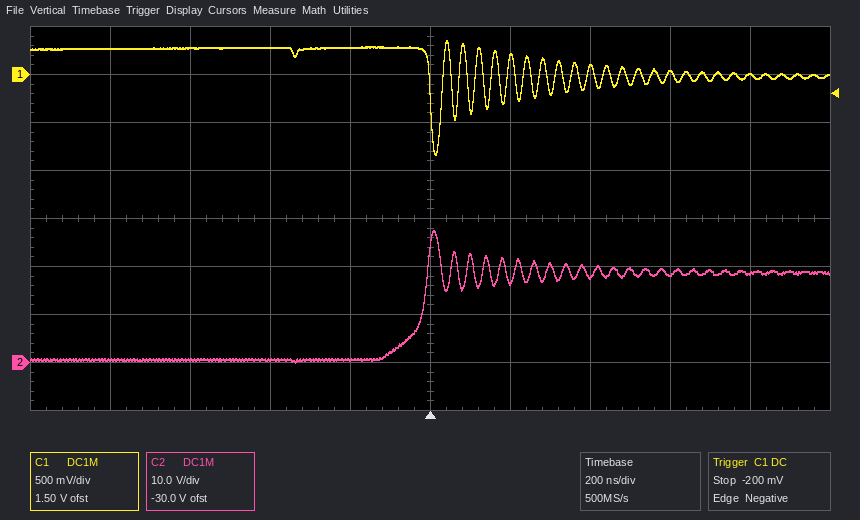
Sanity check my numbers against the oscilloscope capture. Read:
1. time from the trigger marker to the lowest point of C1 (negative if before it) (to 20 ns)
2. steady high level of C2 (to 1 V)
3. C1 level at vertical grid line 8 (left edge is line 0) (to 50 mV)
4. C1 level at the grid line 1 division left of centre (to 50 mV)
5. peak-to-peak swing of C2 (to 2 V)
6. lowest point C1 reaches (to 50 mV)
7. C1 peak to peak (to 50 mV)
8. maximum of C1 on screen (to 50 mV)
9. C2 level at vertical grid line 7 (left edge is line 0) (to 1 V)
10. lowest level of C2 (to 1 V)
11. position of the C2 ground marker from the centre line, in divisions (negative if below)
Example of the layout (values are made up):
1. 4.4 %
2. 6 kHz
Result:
1. +20 ns
2. 19 V
3. 0 mV
4. 300 mV
5. 28 V
6. -850 mV
7. 1.20 V
8. 350 mV
9. 18 V
10. 0 V
11. -3.0 div
